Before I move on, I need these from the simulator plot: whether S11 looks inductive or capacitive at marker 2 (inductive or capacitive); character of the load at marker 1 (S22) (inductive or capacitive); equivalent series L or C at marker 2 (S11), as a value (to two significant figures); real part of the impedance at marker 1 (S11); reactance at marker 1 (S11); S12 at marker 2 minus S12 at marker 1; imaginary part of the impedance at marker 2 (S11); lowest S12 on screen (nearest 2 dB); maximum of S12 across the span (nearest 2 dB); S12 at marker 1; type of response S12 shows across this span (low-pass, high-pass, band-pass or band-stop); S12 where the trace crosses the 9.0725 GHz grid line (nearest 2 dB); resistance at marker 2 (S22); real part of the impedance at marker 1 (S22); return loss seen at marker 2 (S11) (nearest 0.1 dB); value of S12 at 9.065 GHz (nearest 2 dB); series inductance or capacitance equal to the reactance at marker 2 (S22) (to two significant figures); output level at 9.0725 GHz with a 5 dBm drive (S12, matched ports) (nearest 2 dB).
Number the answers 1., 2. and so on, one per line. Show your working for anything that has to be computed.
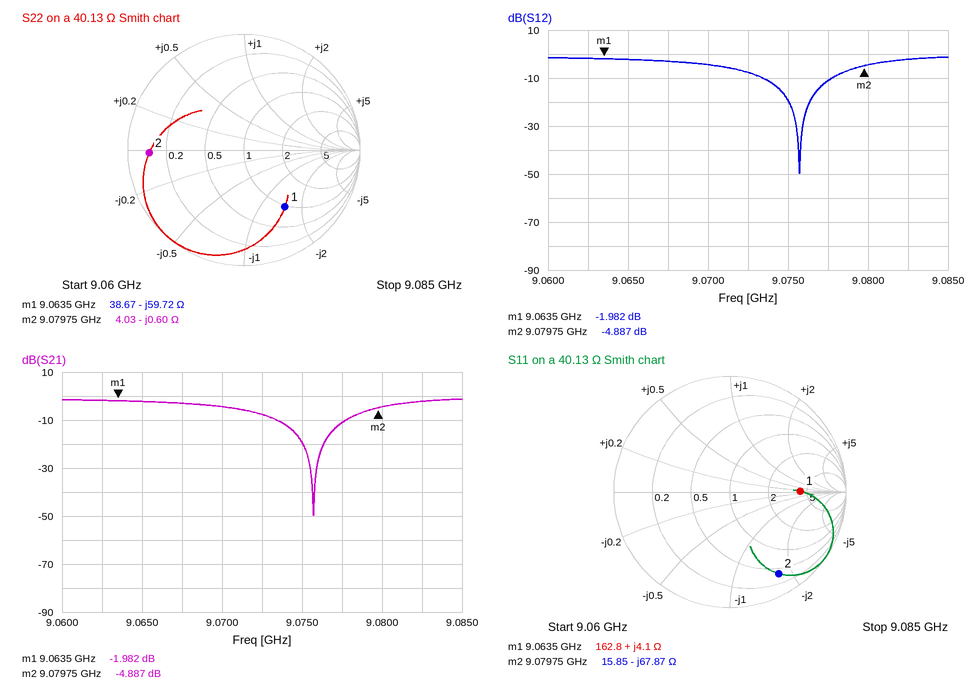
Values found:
1. capacitive
2. capacitive
3. C = 1/(2π × 9.07975 GHz × 67.87 Ω) ≈ 258 fF, so 260 fF to two significant figures
4. 162.8 Ω
5. +4.1 Ω
6. -4.887 − (-1.982) = -2.905 dB
7. -67.87 Ω
8. -50 dB
9. -2 dB
10. -1.982 dB
11. band-stop
12. -8 dB
13. 4.03 Ω
14. 38.67 Ω
15. 1.7 dB
16. -2 dB
17. C = 1/(2π × 9.07975 GHz × 0.6 Ω) ≈ 29 pF
18. 5 dBm + (-8 dB) = -2 dBm
